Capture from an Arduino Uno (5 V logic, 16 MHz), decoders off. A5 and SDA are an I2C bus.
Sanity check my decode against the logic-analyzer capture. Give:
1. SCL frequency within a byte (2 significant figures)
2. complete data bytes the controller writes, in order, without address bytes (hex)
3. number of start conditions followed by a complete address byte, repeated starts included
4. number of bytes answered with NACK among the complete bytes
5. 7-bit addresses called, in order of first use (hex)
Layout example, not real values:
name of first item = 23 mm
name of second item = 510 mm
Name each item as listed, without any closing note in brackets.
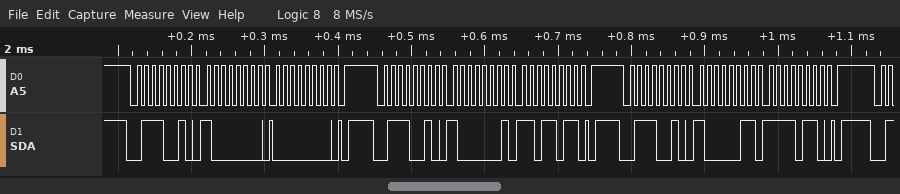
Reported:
SCL frequency within a byte = 100 kHz
complete data bytes the controller writes, in order, without address bytes = 80 00 81 DB 83 F6
number of start conditions followed by a complete address byte, repeated starts included = 3
number of bytes answered with NACK among the complete bytes = 0
7-bit addresses called, in order of first use = 0x39
